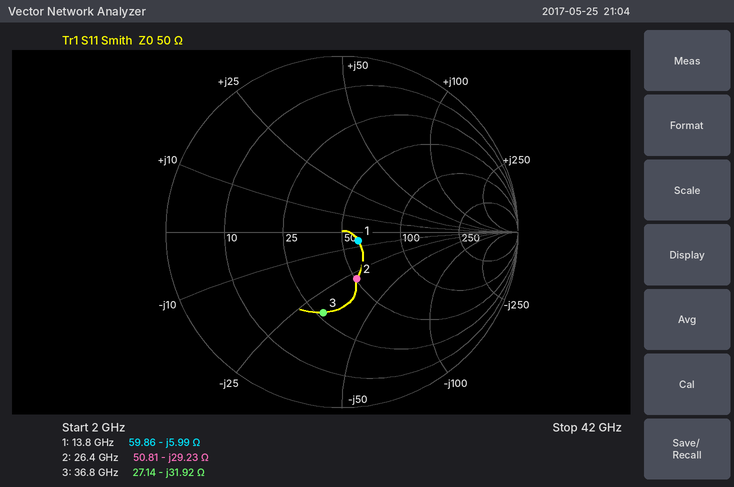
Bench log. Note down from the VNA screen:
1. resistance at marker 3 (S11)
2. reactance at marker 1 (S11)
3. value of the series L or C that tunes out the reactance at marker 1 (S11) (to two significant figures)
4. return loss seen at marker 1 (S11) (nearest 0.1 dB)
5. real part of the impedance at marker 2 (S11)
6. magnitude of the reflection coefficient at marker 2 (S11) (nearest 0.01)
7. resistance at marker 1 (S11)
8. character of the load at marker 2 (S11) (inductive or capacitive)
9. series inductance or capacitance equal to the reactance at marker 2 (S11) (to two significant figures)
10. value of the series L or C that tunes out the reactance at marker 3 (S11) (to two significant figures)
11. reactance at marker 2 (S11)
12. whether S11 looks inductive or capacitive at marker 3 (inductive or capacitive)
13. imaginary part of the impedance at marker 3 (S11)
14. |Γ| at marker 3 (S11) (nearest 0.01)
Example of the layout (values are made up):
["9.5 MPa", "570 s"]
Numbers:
["27.14 Ω", "-5.99 Ω", "69 pH", "19.6 dB", "50.81 Ω", "0.28", "59.86 Ω", "capacitive", "210 fF", "140 pH", "-29.23 Ω", "capacitive", "-31.92 Ω", "0.47"]
